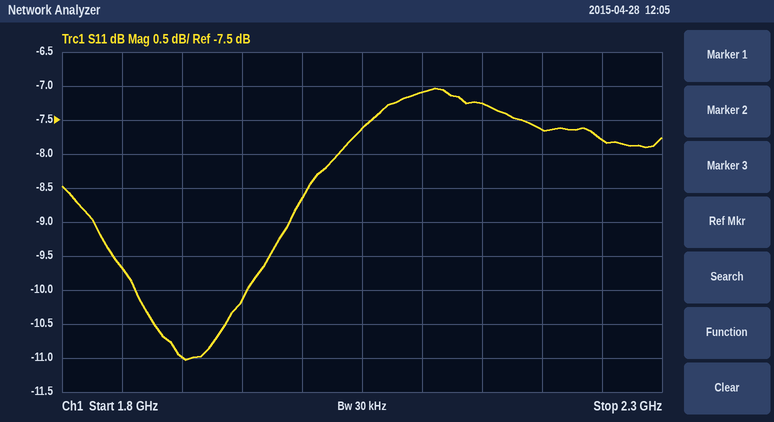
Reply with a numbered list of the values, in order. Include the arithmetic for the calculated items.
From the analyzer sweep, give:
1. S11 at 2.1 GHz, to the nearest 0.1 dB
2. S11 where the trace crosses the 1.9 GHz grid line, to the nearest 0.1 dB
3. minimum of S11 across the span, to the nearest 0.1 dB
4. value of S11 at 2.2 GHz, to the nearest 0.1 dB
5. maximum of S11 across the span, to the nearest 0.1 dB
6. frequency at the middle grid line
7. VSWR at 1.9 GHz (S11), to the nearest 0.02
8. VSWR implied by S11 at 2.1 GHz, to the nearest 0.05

1. -7.1 dB
2. -11.0 dB
3. -11.0 dB
4. -7.6 dB
5. -7.0 dB
6. 2.05 GHz
7. |Γ| = 10^(-11/20) = 0.2818; VSWR = (1 + 0.2818)/(1 − 0.2818) ≈ 1.78
8. |Γ| = 10^(-7.1/20) = 0.4416; VSWR = (1 + 0.4416)/(1 − 0.4416) ≈ 2.58, so 2.60 to the nearest 0.05
